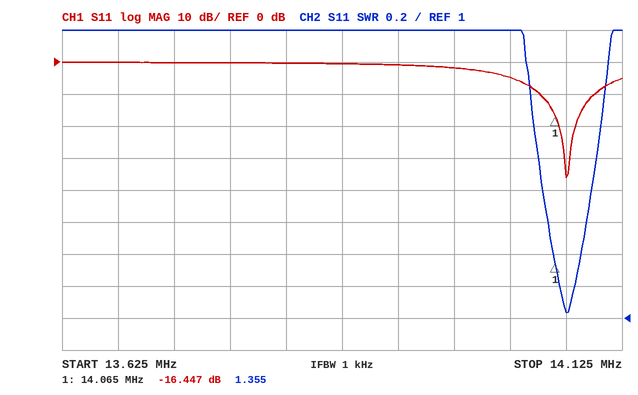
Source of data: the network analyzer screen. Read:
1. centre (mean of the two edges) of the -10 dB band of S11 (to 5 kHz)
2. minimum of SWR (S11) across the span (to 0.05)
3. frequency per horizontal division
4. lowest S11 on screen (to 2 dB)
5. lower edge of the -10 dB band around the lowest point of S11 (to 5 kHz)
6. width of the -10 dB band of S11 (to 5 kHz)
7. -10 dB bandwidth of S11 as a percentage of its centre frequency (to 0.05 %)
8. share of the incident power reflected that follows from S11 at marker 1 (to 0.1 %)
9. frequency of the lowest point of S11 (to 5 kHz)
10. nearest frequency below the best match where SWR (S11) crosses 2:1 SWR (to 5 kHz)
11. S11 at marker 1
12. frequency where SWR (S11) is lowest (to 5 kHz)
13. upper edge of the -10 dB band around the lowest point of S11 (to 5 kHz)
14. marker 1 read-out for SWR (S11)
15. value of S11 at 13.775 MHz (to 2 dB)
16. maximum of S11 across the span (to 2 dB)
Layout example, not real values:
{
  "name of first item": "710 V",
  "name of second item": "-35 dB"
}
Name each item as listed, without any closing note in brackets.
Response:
{
  "centre (mean of the two edges) of the -10 dB band of S11": "14.075 MHz",
  "minimum of SWR (S11) across the span": "1.05",
  "frequency per horizontal division": "50 kHz",
  "lowest S11 on screen": "-36 dB",
  "lower edge of the -10 dB band around the lowest point of S11": "14.050 MHz",
  "width of the -10 dB band of S11": "50 kHz",
  "-10 dB bandwidth of S11 as a percentage of its centre frequency": "0.35 %",
  "share of the incident power reflected that follows from S11 at marker 1": "2.3 %",
  "frequency of the lowest point of S11": "14.075 MHz",
  "nearest frequency below the best match where SWR (S11) crosses 2:1 SWR": "14.050 MHz",
  "S11 at marker 1": "-16.447 dB",
  "frequency where SWR (S11) is lowest": "14.075 MHz",
  "upper edge of the -10 dB band around the lowest point of S11": "14.100 MHz",
  "marker 1 read-out for SWR": "1.355",
  "value of S11 at 13.775 MHz": "0 dB",
  "maximum of S11 across the span": "0 dB"
}
